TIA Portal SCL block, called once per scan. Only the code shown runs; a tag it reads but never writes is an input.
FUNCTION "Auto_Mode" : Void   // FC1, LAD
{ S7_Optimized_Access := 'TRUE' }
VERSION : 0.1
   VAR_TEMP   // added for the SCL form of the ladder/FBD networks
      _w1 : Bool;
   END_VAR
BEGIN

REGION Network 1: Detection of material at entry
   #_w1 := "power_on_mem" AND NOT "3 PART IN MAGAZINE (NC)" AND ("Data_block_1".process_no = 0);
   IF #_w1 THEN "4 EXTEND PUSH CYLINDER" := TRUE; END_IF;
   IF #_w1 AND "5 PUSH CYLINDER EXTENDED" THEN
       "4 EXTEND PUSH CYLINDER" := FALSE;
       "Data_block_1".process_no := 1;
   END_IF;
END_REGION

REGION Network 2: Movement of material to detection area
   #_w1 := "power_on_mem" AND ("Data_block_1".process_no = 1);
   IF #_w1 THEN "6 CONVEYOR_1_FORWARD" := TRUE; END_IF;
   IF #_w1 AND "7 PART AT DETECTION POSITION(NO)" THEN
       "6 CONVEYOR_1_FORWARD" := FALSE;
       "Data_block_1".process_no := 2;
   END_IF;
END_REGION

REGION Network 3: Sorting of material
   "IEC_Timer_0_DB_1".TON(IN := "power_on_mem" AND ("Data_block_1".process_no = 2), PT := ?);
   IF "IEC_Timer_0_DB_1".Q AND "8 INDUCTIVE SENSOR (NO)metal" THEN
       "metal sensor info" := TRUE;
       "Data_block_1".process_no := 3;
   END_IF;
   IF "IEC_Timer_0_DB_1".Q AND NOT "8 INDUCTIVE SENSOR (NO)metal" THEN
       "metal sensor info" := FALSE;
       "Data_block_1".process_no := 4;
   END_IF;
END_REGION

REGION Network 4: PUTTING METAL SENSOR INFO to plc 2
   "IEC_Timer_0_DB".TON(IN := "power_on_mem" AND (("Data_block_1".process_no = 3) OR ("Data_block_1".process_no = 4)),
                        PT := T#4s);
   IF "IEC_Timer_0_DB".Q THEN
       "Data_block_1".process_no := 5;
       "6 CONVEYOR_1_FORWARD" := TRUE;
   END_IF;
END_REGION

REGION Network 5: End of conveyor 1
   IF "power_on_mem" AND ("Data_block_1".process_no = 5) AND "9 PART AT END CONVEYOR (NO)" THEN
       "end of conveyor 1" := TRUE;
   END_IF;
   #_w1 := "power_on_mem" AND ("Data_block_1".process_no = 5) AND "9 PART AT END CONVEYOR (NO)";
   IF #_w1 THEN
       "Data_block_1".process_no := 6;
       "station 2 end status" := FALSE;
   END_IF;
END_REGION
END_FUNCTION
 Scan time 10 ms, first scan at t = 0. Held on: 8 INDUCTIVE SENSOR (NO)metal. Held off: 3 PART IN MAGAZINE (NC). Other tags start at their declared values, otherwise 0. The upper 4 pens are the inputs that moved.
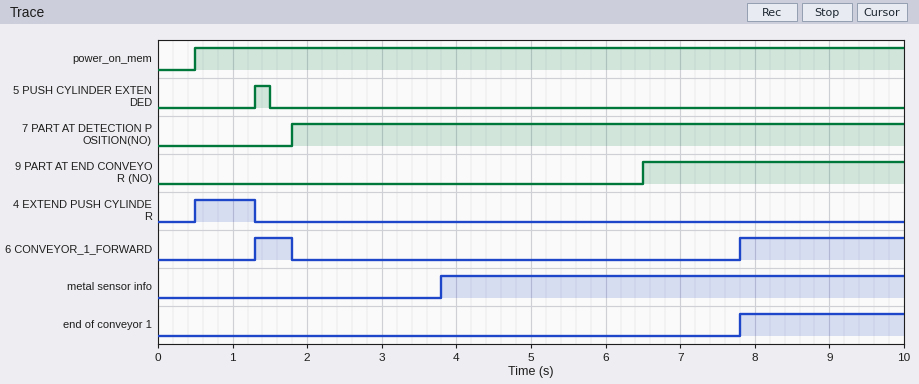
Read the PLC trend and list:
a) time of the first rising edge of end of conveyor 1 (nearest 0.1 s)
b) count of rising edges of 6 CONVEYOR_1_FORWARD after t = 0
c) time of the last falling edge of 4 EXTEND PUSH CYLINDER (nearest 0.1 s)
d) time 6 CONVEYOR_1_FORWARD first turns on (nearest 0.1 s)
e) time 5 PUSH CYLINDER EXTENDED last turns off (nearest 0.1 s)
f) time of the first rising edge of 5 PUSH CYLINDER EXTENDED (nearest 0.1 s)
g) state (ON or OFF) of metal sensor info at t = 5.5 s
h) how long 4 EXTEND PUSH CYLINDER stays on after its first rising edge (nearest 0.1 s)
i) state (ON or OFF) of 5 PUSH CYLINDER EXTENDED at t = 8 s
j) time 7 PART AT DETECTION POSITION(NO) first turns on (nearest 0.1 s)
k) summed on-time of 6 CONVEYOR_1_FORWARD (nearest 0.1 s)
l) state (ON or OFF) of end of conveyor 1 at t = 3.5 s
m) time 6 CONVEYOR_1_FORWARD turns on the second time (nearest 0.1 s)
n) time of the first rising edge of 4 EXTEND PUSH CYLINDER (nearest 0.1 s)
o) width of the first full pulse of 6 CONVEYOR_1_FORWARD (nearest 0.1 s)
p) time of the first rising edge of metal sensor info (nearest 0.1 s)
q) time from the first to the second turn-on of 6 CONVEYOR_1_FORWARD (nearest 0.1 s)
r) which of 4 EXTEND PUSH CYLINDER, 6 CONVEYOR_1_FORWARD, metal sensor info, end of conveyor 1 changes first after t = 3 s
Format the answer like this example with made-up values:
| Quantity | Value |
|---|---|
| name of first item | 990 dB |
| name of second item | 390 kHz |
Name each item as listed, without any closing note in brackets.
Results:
| Quantity | Value |
|---|---|
| time of the first rising edge of end of conveyor 1 | 7.8 s |
| count of rising edges of 6 CONVEYOR_1_FORWARD after t = 0 | 2 |
| time of the last falling edge of 4 EXTEND PUSH CYLINDER | 1.3 s |
| time 6 CONVEYOR_1_FORWARD first turns on | 1.3 s |
| time 5 PUSH CYLINDER EXTENDED last turns off | 1.5 s |
| time of the first rising edge of 5 PUSH CYLINDER EXTENDED | 1.3 s |
| state (ON or OFF) of metal sensor info at t = 5.5 s | ON |
| how long 4 EXTEND PUSH CYLINDER stays on after its first rising edge | 0.8 s |
| state (ON or OFF) of 5 PUSH CYLINDER EXTENDED at t = 8 s | OFF |
| time 7 PART AT DETECTION POSITION(NO) first turns on | 1.8 s |
| summed on-time of 6 CONVEYOR_1_FORWARD | 2.7 s |
| state (ON or OFF) of end of conveyor 1 at t = 3.5 s | OFF |
| time 6 CONVEYOR_1_FORWARD turns on the second time | 7.8 s |
| time of the first rising edge of 4 EXTEND PUSH CYLINDER | 0.5 s |
| width of the first full pulse of 6 CONVEYOR_1_FORWARD | 0.5 s |
| time of the first rising edge of metal sensor info | 3.8 s |
| time from the first to the second turn-on of 6 CONVEYOR_1_FORWARD | 6.5 s |
| which of 4 EXTEND PUSH CYLINDER, 6 CONVEYOR_1_FORWARD, metal sensor info, end of conveyor 1 changes first after t = 3 s | metal sensor info |
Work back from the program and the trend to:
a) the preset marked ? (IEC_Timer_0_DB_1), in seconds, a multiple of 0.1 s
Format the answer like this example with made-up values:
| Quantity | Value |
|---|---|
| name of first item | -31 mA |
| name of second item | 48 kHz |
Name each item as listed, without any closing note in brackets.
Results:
| Quantity | Value |
|---|---|
| the preset marked ? (IEC_Timer_0_DB_1), in seconds, a multiple of 0.1 s | 2.0 s |
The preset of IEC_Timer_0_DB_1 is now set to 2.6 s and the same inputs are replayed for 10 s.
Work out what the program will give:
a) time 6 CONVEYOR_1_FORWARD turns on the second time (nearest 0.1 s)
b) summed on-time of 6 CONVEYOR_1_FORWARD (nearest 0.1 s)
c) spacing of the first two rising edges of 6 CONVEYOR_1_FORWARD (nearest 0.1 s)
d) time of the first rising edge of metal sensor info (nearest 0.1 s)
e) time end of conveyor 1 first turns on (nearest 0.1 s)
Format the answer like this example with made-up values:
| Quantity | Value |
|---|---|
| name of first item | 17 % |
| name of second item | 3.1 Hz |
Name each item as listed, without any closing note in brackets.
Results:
| Quantity | Value |
|---|---|
| time 6 CONVEYOR_1_FORWARD turns on the second time | 8.4 s |
| summed on-time of 6 CONVEYOR_1_FORWARD | 2.1 s |
| spacing of the first two rising edges of 6 CONVEYOR_1_FORWARD | 7.1 s |
| time of the first rising edge of metal sensor info | 4.4 s |
| time end of conveyor 1 first turns on | 8.4 s |
